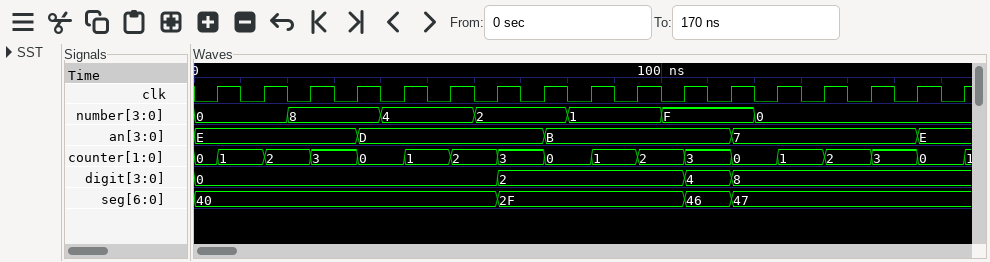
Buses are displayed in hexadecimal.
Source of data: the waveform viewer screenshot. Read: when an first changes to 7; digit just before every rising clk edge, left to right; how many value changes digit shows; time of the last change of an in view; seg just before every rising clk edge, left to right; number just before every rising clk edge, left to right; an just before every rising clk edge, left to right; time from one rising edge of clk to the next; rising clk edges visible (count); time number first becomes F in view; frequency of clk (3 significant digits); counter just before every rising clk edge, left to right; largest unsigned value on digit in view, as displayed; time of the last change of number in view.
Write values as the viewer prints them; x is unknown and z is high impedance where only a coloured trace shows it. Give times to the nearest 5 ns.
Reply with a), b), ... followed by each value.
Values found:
a) 115 ns
b) 0, 0, 0, 0, 0, 0, 0, 2, 2, 2, 2, 4, 8, 8, 8, 8, 8
c) 3
d) 155 ns
e) 40, 40, 40, 40, 40, 40, 40, 2F, 2F, 2F, 2F, 46, 47, 47, 47, 47, 47
f) 0, 0, 8, 8, 4, 4, 2, 2, 1, 1, F, F, 0, 0, 0, 0, 0
g) E, E, E, E, D, D, D, D, B, B, B, B, 7, 7, 7, 7, E
h) 10 ns
i) 17
j) 100 ns
k) 100 MHz
l) 0, 1, 2, 3, 0, 1, 2, 3, 0, 1, 2, 3, 0, 1, 2, 3, 0
m) 8
n) 120 ns
